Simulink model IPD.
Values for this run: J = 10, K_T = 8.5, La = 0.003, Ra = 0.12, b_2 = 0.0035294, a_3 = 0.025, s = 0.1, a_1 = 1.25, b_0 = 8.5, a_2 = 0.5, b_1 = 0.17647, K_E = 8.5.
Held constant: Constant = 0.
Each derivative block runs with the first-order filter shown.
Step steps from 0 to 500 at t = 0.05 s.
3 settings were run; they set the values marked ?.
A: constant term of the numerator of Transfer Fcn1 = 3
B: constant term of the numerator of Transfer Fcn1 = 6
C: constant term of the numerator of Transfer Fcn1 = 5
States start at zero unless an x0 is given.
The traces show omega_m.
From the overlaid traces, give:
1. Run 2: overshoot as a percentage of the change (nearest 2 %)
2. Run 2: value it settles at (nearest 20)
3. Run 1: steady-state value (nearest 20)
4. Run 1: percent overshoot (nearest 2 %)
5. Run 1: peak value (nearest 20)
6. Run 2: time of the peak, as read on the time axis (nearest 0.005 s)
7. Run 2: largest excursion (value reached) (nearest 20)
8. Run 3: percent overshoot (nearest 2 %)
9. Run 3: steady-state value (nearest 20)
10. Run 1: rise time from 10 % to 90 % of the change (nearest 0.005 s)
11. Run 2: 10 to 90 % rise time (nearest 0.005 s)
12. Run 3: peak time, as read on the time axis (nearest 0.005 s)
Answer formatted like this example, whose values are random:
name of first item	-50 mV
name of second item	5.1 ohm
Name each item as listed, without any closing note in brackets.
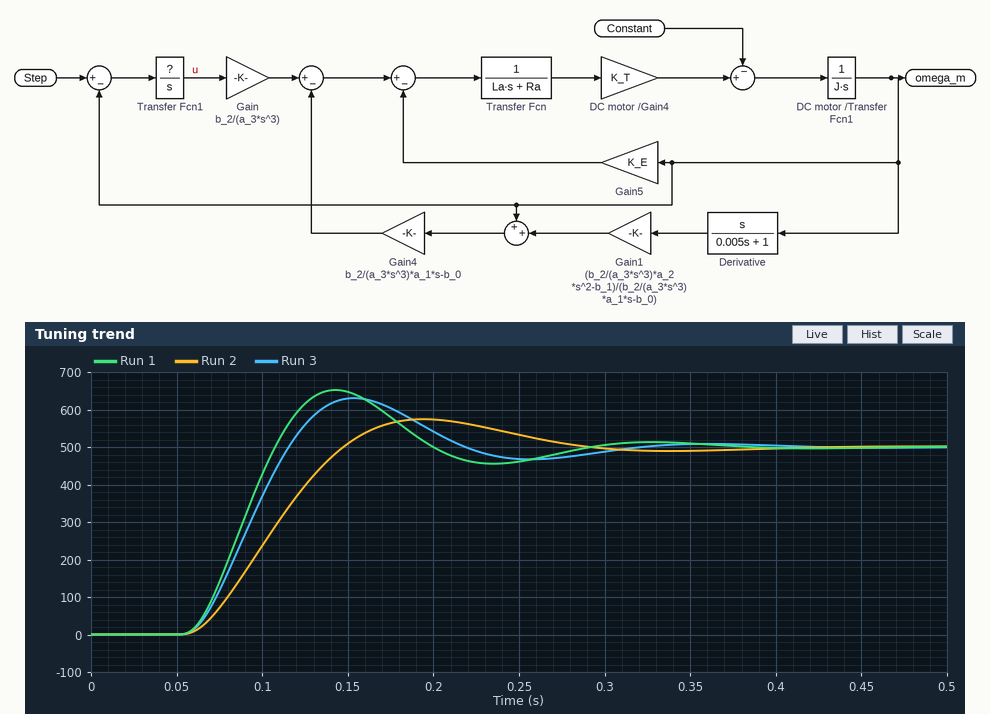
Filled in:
Run 2: overshoot as a percentage of the change	14 %
Run 2: value it settles at	500
Run 1: steady-state value	500
Run 1: percent overshoot	30 %
Run 1: peak value	660
Run 2: time of the peak, as read on the time axis	0.195 s
Run 2: largest excursion (value reached)	580
Run 3: percent overshoot	26 %
Run 3: steady-state value	500
Run 1: rise time from 10 % to 90 % of the change	0.035 s
Run 2: 10 to 90 % rise time	0.065 s
Run 3: peak time, as read on the time axis	0.155 s
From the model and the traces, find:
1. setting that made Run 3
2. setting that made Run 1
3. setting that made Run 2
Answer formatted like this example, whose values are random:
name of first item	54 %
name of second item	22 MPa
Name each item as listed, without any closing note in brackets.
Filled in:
setting that made Run 3	C
setting that made Run 1	B
setting that made Run 2	A
